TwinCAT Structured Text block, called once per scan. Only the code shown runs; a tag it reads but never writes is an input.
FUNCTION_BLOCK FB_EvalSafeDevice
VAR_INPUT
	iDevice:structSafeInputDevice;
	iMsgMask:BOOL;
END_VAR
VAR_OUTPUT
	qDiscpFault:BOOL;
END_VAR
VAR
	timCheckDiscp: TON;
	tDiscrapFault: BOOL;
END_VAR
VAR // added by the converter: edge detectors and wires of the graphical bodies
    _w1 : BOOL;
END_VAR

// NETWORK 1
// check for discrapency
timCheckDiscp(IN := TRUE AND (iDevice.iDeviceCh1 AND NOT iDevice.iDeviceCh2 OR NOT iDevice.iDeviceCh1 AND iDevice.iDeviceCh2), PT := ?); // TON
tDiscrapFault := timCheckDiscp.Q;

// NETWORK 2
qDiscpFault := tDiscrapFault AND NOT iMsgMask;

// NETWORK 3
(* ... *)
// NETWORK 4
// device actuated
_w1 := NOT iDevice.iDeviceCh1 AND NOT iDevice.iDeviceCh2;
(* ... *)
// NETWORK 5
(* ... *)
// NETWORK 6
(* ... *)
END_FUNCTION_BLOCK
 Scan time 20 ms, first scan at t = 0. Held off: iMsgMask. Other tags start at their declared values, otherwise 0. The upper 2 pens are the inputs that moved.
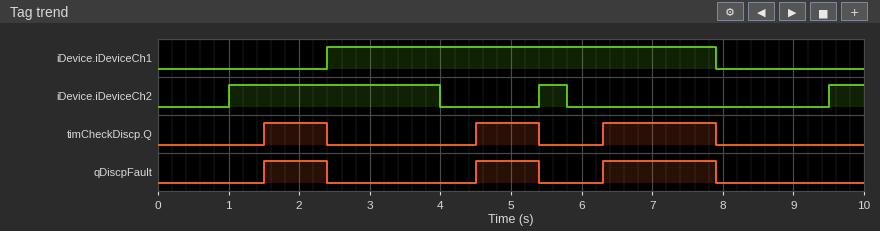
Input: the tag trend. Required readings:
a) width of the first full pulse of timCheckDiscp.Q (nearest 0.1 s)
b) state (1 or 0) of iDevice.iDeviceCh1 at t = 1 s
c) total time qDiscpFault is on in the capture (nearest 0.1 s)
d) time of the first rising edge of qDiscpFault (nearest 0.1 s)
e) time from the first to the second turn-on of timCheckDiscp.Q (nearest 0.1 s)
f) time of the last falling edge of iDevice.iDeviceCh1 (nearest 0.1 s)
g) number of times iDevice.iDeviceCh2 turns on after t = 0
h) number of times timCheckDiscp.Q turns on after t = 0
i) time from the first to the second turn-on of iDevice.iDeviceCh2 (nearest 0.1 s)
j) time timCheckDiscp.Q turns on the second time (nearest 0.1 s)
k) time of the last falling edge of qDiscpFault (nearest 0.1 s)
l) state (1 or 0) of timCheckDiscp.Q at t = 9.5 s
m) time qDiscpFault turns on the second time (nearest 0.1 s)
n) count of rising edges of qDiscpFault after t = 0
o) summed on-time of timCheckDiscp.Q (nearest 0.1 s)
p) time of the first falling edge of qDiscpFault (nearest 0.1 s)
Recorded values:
0.9 s
0
3.4 s
1.5 s
3.0 s
7.9 s
3
3
4.4 s
4.5 s
7.9 s
0
4.5 s
3
3.4 s
2.4 s
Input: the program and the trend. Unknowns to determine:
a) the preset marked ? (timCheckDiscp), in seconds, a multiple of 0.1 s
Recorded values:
0.5 s
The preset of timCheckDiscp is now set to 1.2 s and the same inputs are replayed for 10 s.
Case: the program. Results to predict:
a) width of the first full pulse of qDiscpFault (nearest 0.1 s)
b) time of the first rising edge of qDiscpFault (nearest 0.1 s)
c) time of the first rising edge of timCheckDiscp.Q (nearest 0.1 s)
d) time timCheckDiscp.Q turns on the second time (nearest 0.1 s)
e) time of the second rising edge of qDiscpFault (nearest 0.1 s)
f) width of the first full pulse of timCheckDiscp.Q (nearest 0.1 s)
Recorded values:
0.2 s
2.2 s
2.2 s
5.2 s
5.2 s
0.2 s
